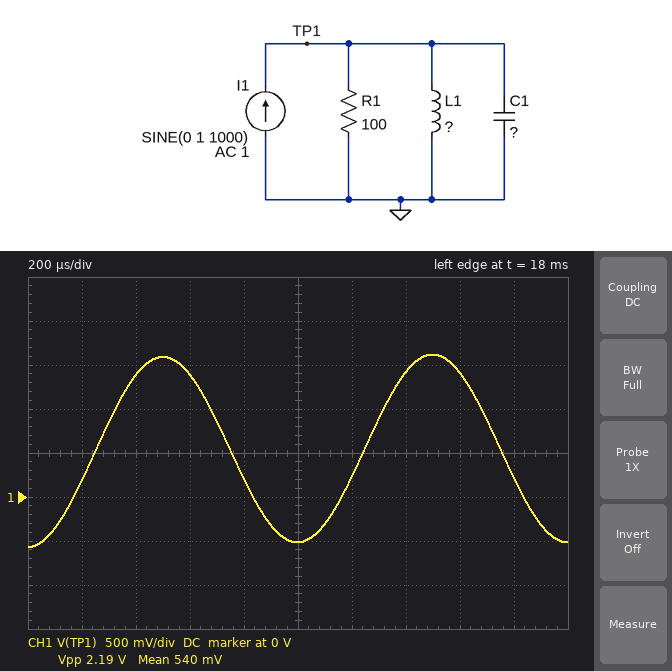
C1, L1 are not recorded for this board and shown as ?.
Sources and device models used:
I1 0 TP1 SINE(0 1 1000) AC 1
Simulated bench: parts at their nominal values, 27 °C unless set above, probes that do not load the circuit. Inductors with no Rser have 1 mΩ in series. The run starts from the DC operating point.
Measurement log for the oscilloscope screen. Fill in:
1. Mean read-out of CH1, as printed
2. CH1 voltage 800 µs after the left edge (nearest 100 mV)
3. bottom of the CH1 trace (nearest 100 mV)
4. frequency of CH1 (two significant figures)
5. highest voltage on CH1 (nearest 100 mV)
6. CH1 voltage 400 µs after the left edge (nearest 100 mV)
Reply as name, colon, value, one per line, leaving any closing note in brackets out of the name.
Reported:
Mean read-out of CH1, as printed: 540 mV
CH1 voltage 800 µs after the left edge: 200 mV
bottom of the CH1 trace: -600 mV
frequency of CH1: 1.0 kHz
highest voltage on CH1: 1.6 V
CH1 voltage 400 µs after the left edge: 1.4 V
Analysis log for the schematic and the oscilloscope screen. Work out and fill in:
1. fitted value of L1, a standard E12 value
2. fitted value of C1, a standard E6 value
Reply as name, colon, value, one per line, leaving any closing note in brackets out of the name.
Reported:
fitted value of L1, a standard E12 value: 68 mH
fitted value of C1, a standard E6 value: 150 µF
